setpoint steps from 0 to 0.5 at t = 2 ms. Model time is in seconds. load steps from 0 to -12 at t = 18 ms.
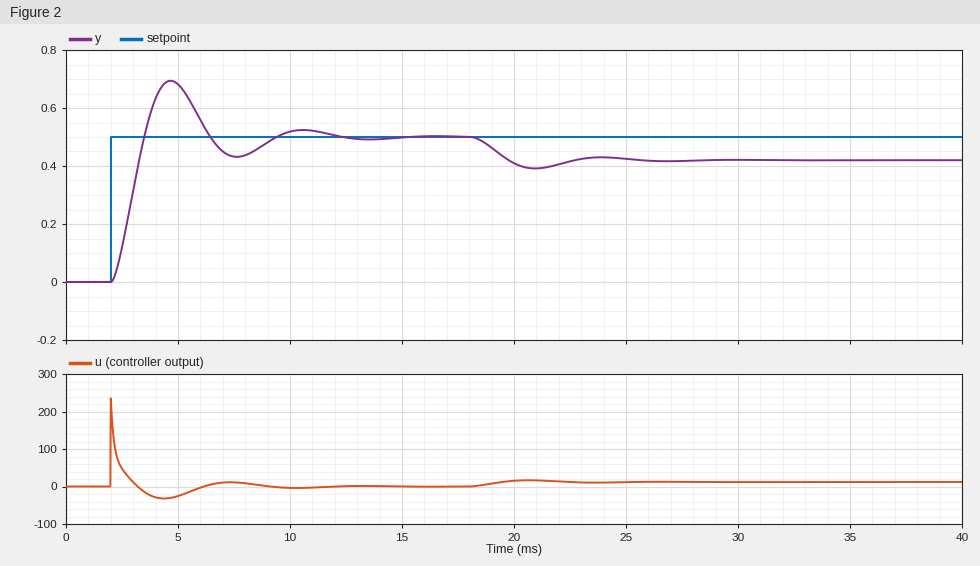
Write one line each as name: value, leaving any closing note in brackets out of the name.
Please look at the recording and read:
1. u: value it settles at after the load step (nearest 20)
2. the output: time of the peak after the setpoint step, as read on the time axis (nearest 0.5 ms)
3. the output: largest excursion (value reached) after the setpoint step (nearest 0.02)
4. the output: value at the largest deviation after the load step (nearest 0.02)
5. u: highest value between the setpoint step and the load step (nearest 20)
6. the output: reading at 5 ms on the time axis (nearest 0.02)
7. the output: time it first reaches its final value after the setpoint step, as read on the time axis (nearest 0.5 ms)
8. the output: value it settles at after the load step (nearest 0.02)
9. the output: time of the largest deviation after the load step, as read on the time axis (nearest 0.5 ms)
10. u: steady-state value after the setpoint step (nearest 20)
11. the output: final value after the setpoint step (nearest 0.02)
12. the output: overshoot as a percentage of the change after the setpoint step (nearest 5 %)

u: value it settles at after the load step: 20
the output: time of the peak after the setpoint step, as read on the time axis: 4.5 ms
the output: largest excursion (value reached) after the setpoint step: 0.70
the output: value at the largest deviation after the load step: 0.40
u: highest value between the setpoint step and the load step: 240
the output: reading at 5 ms on the time axis: 0.68
the output: time it first reaches its final value after the setpoint step, as read on the time axis: 3.5 ms
the output: value it settles at after the load step: 0.42
the output: time of the largest deviation after the load step, as read on the time axis: 21.0 ms
u: steady-state value after the setpoint step: 0
the output: final value after the setpoint step: 0.50
the output: overshoot as a percentage of the change after the setpoint step: 40 %
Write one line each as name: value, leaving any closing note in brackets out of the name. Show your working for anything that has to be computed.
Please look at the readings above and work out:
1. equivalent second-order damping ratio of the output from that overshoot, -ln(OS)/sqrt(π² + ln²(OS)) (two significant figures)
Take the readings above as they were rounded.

equivalent second-order damping ratio of the output from that overshoot, -ln(OS)/sqrt(π² + ln²(OS)): ln(0.4) = -0.916; 0.916 / sqrt(9.870 + 0.840) = 0.28
